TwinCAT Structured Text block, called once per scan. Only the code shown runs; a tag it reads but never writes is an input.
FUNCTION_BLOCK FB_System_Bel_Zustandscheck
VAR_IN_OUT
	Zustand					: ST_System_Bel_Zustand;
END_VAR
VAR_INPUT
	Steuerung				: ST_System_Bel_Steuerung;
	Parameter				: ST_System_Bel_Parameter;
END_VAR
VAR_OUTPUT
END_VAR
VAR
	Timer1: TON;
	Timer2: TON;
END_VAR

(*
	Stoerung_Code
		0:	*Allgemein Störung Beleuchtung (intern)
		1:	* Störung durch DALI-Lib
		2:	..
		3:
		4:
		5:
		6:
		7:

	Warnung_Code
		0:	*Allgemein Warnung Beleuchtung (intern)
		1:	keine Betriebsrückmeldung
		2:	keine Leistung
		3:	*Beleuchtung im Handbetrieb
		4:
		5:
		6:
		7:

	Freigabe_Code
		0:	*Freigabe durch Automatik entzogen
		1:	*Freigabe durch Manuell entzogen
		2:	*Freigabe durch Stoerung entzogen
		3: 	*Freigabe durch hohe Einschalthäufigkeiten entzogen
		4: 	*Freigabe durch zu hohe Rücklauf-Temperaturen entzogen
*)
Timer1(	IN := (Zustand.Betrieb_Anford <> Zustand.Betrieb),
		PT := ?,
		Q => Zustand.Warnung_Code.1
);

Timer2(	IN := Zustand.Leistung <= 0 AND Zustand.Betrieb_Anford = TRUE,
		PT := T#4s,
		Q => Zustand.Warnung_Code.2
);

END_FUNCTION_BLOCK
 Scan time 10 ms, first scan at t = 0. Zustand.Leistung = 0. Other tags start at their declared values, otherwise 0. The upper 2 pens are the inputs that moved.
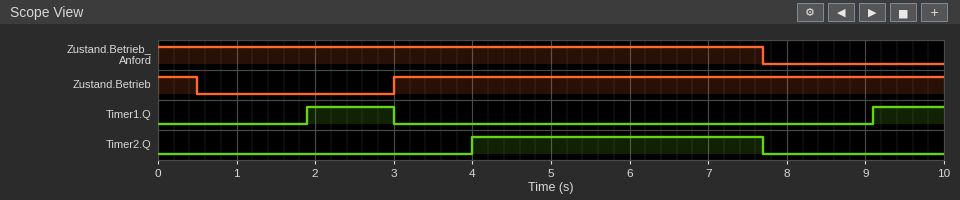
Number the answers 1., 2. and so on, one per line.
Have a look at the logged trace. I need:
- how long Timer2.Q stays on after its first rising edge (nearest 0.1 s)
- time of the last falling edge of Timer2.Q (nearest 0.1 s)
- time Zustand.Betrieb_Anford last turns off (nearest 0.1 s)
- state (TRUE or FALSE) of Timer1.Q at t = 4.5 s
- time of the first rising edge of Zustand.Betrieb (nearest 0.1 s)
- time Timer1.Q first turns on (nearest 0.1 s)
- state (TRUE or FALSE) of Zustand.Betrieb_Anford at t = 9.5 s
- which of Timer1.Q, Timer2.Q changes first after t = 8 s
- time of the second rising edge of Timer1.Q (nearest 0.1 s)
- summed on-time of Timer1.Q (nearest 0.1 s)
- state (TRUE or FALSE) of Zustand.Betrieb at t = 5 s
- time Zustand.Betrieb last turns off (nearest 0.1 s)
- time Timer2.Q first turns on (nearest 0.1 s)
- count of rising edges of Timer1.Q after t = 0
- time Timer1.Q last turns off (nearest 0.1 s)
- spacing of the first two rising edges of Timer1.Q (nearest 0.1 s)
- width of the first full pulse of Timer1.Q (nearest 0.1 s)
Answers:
1. 3.7 s
2. 7.7 s
3. 7.7 s
4. FALSE
5. 3.0 s
6. 1.9 s
7. FALSE
8. Timer1.Q
9. 9.1 s
10. 2.0 s
11. TRUE
12. 0.5 s
13. 4.0 s
14. 2
15. 3.0 s
16. 7.2 s
17. 1.1 s
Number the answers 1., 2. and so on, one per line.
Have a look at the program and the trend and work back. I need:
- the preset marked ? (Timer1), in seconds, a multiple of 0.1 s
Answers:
1. 1.4 s
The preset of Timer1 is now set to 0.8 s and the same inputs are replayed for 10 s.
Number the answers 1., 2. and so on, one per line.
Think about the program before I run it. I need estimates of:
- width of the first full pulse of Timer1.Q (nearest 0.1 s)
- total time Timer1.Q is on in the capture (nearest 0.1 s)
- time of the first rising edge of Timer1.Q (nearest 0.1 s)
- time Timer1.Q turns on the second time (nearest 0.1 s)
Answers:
1. 1.7 s
2. 3.2 s
3. 1.3 s
4. 8.5 s
